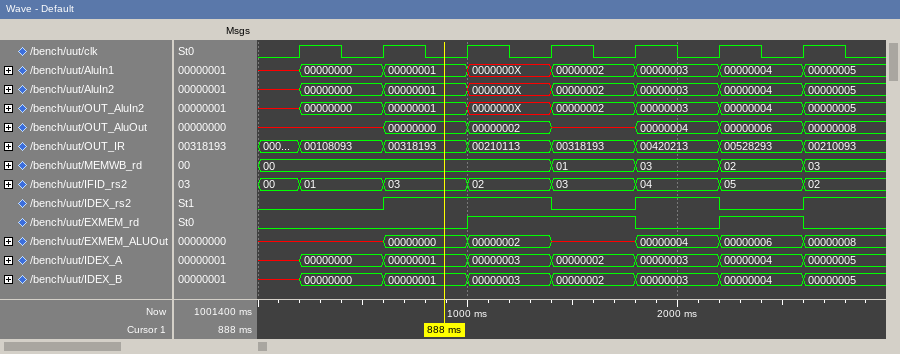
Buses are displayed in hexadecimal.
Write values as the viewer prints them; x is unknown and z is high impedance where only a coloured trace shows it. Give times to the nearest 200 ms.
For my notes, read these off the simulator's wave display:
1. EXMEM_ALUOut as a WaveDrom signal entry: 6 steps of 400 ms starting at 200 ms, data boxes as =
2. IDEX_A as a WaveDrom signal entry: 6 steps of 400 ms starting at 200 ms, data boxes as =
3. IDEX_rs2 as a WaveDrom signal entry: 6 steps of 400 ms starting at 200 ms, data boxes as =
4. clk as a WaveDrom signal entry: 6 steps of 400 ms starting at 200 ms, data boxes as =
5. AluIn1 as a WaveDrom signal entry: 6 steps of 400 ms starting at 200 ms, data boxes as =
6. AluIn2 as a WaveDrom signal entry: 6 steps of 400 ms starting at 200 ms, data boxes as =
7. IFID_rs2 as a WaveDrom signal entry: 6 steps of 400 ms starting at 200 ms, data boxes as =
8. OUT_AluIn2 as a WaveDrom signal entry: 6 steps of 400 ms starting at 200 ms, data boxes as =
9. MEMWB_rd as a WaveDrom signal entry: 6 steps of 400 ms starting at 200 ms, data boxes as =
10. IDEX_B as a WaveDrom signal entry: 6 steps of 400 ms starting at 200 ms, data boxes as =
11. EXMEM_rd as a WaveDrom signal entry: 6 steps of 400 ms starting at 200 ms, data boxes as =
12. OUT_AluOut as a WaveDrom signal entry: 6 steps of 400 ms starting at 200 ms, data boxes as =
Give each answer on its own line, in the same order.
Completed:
{name: 'EXMEM_ALUOut', wave: 'x==x==', data: '00000000 00000002 00000004 00000006'}
{name: 'IDEX_A', wave: '======', data: '00000000 00000001 00000003 00000002 00000003 00000004'}
{name: 'IDEX_rs2', wave: '01.010'}
{name: 'clk', wave: 'p.....'}
{name: 'AluIn1', wave: '======', data: '00000000 00000001 0000000X 00000002 00000003 00000004'}
{name: 'AluIn2', wave: '======', data: '00000000 00000001 0000000X 00000002 00000003 00000004'}
{name: 'IFID_rs2', wave: '======', data: '01 03 02 03 04 05'}
{name: 'OUT_AluIn2', wave: '======', data: '00000000 00000001 0000000X 00000002 00000003 00000004'}
{name: 'MEMWB_rd', wave: '=..===', data: '00 01 03 02'}
{name: 'IDEX_B', wave: '======', data: '00000000 00000001 00000003 00000002 00000003 00000004'}
{name: 'EXMEM_rd', wave: '0.1.01'}
{name: 'OUT_AluOut', wave: 'x==x==', data: '00000000 00000002 00000004 00000006'}
